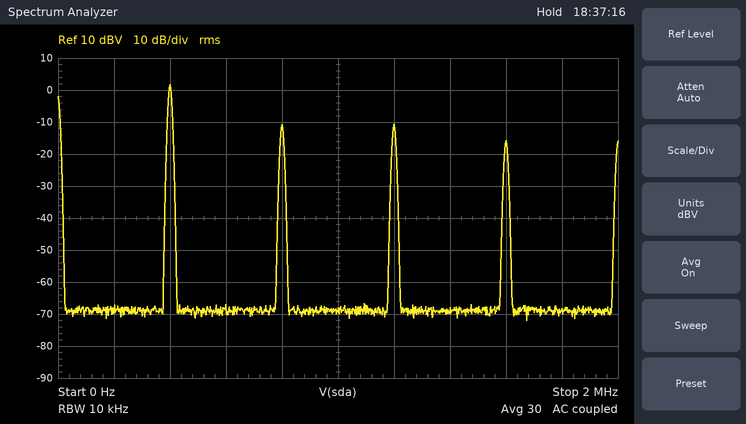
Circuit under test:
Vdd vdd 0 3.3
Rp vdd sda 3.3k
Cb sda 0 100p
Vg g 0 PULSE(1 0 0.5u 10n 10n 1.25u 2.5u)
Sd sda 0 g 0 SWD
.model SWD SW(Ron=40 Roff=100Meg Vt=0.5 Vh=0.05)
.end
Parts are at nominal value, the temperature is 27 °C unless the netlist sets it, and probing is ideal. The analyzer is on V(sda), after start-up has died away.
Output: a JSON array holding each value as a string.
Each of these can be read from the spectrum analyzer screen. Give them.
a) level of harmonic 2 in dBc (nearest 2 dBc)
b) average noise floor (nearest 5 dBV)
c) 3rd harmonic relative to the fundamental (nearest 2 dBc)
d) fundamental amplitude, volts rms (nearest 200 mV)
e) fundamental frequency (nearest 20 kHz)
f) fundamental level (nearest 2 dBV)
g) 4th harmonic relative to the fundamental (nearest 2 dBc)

["-12 dBc", "-70 dBV", "-12 dBc", "1.2 V", "400 kHz", "2 dBV", "-18 dBc"]
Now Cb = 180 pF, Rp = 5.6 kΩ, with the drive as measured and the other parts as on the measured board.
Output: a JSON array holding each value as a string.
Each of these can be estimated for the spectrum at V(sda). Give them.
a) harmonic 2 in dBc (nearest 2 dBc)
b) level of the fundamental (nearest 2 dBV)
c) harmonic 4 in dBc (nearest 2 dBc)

["-10 dBc", "-2 dBV", "-16 dBc"]
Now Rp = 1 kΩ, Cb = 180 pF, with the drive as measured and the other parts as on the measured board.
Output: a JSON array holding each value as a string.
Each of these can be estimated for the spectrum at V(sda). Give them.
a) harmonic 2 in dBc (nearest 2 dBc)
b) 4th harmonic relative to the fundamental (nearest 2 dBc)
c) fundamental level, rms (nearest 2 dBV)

["-16 dBc", "-20 dBc", "2 dBV"]
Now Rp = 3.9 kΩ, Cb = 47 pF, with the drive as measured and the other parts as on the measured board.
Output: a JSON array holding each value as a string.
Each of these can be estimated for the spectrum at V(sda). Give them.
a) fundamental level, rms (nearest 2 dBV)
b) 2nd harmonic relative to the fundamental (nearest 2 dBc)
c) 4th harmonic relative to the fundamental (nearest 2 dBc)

["2 dBV", "-16 dBc", "-20 dBc"]
